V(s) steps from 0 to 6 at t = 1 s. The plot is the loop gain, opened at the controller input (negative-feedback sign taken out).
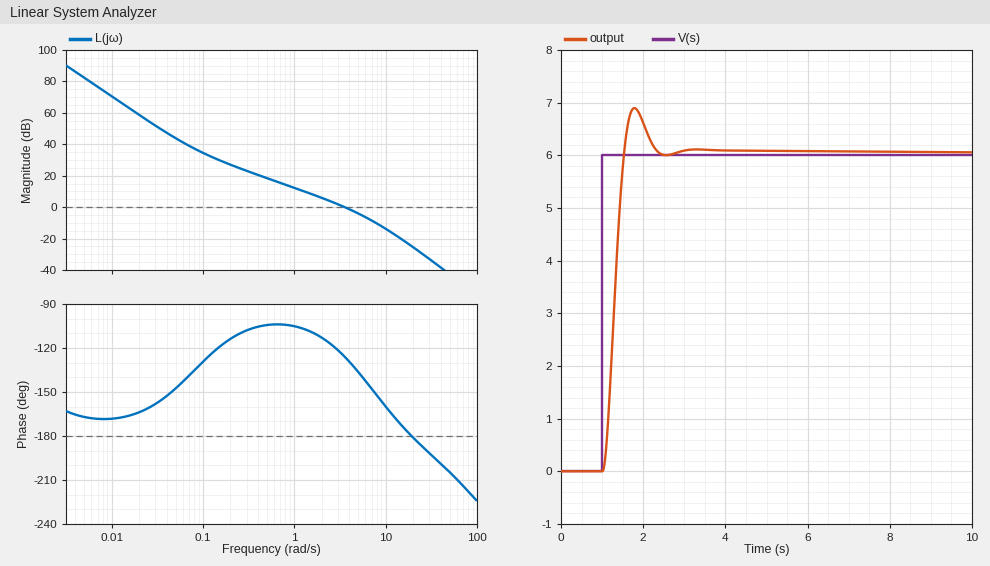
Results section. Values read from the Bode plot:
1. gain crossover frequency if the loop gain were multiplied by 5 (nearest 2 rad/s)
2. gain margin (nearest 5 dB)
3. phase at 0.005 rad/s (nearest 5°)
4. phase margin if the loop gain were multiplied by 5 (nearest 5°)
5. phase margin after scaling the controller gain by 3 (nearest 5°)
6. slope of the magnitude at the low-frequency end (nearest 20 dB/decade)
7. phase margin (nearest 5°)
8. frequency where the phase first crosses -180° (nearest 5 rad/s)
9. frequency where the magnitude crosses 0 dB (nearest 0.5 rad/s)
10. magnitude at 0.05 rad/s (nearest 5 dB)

10 rad/s
25 dB
-165°
20°
30°
-40 dB/decade
55°
20 rad/s
3.5 rad/s
45 dB
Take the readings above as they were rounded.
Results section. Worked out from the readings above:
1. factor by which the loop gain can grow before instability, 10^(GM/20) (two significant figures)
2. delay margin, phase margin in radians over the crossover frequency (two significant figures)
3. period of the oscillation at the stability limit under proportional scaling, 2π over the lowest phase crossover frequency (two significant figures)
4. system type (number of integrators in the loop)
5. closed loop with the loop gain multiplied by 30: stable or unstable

18
0.27 s
0.31 s
2
unstable
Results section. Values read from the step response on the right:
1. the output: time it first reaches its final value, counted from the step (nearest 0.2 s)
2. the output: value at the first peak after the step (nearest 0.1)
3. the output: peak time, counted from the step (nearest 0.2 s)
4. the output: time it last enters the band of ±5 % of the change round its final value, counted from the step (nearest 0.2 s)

0.6 s
6.9
0.8 s
1.2 s
